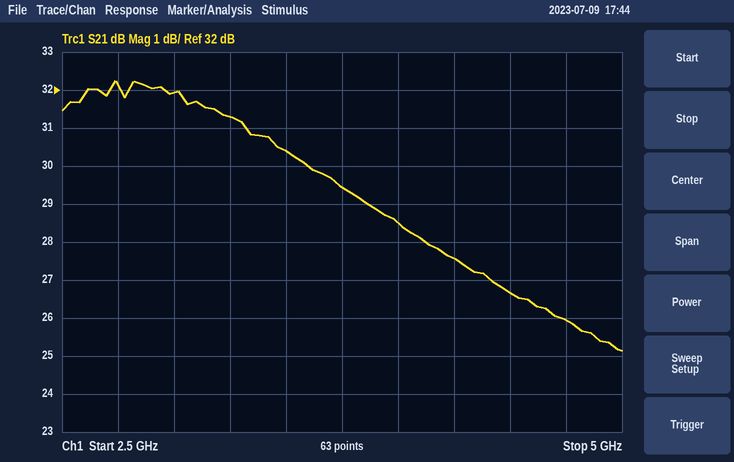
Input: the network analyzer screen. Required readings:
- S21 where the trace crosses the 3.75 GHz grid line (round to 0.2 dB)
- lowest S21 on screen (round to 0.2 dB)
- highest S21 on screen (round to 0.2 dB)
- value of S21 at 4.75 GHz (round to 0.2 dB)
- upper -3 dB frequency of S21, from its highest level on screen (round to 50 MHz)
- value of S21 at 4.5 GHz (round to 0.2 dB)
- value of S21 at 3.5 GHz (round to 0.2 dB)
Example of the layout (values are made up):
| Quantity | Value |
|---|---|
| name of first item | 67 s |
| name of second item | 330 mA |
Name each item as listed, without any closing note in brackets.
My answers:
| Quantity | Value |
|---|---|
| S21 where the trace crosses the 3.75 GHz grid line | 29.4 dB |
| lowest S21 on screen | 25.2 dB |
| highest S21 on screen | 32.2 dB |
| value of S21 at 4.75 GHz | 26.0 dB |
| upper -3 dB frequency of S21, from its highest level on screen | 3.80 GHz |
| value of S21 at 4.5 GHz | 26.6 dB |
| value of S21 at 3.5 GHz | 30.4 dB |
